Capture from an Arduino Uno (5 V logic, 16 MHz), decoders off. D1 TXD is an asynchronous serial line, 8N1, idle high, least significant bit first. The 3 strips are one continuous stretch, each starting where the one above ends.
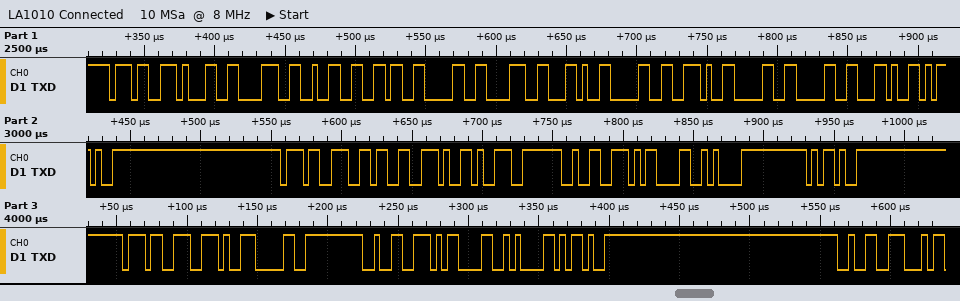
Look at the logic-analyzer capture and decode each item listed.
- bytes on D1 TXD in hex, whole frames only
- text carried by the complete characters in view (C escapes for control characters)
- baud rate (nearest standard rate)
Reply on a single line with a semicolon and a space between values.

0x37 0x31 0x38 0x32 0x36 0x30 0x38 0x2C 0x30 0x2E 0x30 0x30 0x2C 0x2D 0x37 0x36 0x2E 0x39 0x32 0x0D 0x0A 0x2D 0x37 0x2E 0x30 0x32 0x0D 0x0A 0x2D 0x32; "7182608,0.00,-76.92\r\n-7.02\r\n-2"; 250000 baud
